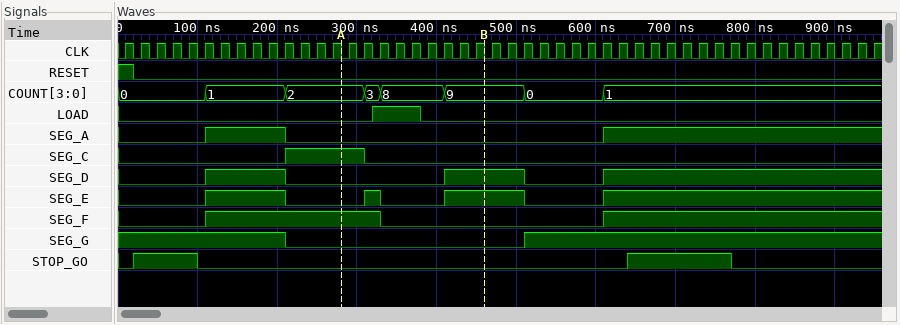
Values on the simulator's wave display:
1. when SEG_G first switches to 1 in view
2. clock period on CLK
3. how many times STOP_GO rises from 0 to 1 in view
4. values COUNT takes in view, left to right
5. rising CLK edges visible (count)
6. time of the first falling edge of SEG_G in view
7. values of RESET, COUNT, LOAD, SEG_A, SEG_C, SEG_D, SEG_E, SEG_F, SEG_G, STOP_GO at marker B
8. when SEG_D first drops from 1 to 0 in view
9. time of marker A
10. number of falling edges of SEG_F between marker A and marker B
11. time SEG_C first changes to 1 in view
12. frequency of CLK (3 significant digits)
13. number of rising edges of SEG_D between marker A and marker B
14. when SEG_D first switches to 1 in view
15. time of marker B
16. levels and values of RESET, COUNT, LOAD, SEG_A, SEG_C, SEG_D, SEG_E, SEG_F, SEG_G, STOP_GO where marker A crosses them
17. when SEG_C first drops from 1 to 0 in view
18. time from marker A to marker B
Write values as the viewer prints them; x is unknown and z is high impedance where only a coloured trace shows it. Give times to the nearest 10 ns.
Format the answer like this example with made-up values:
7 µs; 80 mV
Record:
510 ns; 20 ns; 2; 0, 1, 2, 3, 8, 9, 0, 1; 48; 210 ns; RESET=0, COUNT=9, LOAD=0, SEG_A=0, SEG_C=0, SEG_D=1, SEG_E=1, SEG_F=0, SEG_G=0, STOP_GO=0; 210 ns; 280 ns; 1; 210 ns; 50.0 MHz; 1; 110 ns; 460 ns; RESET=0, COUNT=2, LOAD=0, SEG_A=0, SEG_C=1, SEG_D=0, SEG_E=0, SEG_F=1, SEG_G=0, STOP_GO=0; 310 ns; 180 ns
